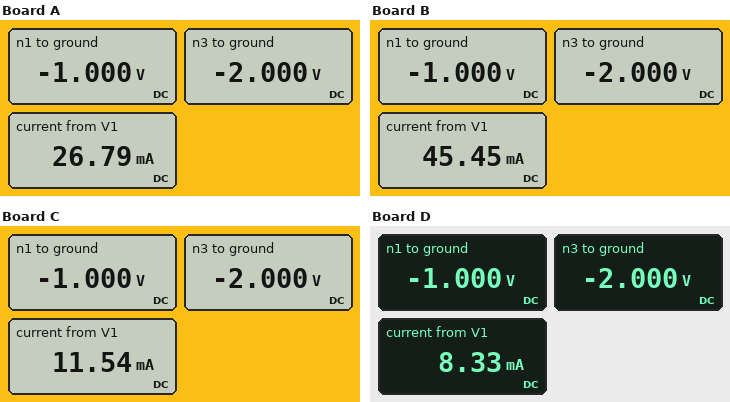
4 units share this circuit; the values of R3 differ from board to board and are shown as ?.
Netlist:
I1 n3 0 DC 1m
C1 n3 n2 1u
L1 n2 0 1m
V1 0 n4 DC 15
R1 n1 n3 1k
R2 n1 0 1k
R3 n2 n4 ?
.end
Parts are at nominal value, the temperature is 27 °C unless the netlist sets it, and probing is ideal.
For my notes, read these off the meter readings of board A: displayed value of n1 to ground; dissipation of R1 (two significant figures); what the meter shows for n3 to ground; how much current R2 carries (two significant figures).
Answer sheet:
-1.000 V
1.0 mW
-2.000 V
1.0 mA
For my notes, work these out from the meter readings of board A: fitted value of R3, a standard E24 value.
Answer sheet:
560 Ω
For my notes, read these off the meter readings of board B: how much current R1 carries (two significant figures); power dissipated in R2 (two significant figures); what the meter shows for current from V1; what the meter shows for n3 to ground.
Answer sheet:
1.0 mA
1.0 mW
45.45 mA
-2.000 V
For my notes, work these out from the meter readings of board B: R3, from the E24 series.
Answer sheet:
330 Ω
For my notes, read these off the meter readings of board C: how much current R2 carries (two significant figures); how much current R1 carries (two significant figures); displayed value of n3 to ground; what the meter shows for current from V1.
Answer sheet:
1.0 mA
1.0 mA
-2.000 V
11.54 mA
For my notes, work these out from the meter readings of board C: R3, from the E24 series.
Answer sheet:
1.3 kΩ
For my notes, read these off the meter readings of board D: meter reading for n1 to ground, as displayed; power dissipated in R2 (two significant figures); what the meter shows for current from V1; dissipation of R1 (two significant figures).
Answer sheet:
-1.000 V
1.0 mW
8.33 mA
1.0 mW
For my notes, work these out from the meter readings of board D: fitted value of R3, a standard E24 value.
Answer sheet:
1.8 kΩ
